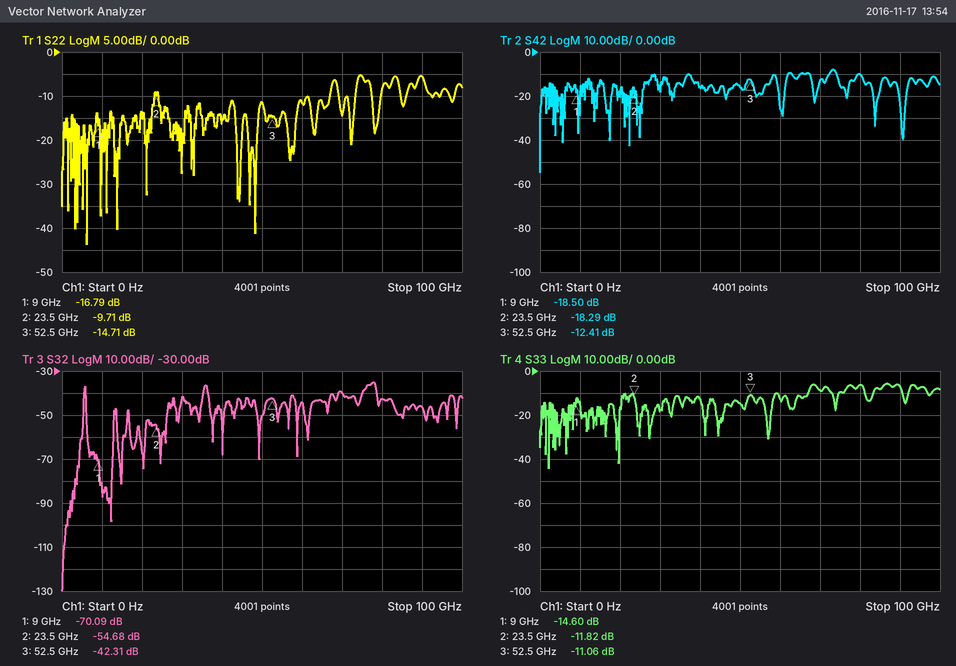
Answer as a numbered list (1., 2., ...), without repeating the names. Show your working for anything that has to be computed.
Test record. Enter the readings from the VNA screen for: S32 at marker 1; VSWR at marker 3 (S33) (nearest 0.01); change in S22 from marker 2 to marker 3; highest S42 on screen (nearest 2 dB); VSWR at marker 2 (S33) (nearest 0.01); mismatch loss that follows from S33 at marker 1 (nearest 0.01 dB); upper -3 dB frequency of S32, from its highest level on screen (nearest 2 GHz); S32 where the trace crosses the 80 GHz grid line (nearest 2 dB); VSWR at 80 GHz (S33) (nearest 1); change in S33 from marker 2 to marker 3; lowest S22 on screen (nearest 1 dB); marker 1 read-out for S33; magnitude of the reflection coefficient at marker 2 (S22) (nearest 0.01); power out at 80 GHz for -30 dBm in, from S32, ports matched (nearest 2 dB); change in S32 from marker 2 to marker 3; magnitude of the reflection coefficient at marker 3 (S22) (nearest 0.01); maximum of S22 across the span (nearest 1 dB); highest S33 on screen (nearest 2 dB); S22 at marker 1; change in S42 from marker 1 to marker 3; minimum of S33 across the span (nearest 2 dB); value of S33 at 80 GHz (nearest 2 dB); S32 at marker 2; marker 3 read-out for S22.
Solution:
1. -70.09 dB
2. (1 + 0.2799)/(1 − 0.2799) ≈ 1.78
3. -14.71 − (-9.71) = -5.00 dB
4. -8 dB
5. (1 + 0.2564)/(1 − 0.2564) ≈ 1.69
6. −10 log10(1 − 10^(-14.6/10)) ≈ 0.15 dB
7. 78 GHz
8. -42 dB
9. |Γ| = 10^(-6/20) = 0.5012; VSWR = (1 + 0.5012)/(1 − 0.5012) ≈ 3
10. -11.06 − (-11.82) = 0.76 dB
11. -44 dB
12. -14.60 dB
13. 10^(-9.71/20) ≈ 0.33
14. -30 dBm + (-42 dB) = -72 dBm
15. -42.31 − (-54.68) = 12.37 dB
16. 10^(-14.71/20) ≈ 0.18
17. -5 dB
18. -6 dB
19. -16.79 dB
20. -12.41 − (-18.5) = 6.09 dB
21. -44 dB
22. -6 dB
23. -54.68 dB
24. -14.71 dB
